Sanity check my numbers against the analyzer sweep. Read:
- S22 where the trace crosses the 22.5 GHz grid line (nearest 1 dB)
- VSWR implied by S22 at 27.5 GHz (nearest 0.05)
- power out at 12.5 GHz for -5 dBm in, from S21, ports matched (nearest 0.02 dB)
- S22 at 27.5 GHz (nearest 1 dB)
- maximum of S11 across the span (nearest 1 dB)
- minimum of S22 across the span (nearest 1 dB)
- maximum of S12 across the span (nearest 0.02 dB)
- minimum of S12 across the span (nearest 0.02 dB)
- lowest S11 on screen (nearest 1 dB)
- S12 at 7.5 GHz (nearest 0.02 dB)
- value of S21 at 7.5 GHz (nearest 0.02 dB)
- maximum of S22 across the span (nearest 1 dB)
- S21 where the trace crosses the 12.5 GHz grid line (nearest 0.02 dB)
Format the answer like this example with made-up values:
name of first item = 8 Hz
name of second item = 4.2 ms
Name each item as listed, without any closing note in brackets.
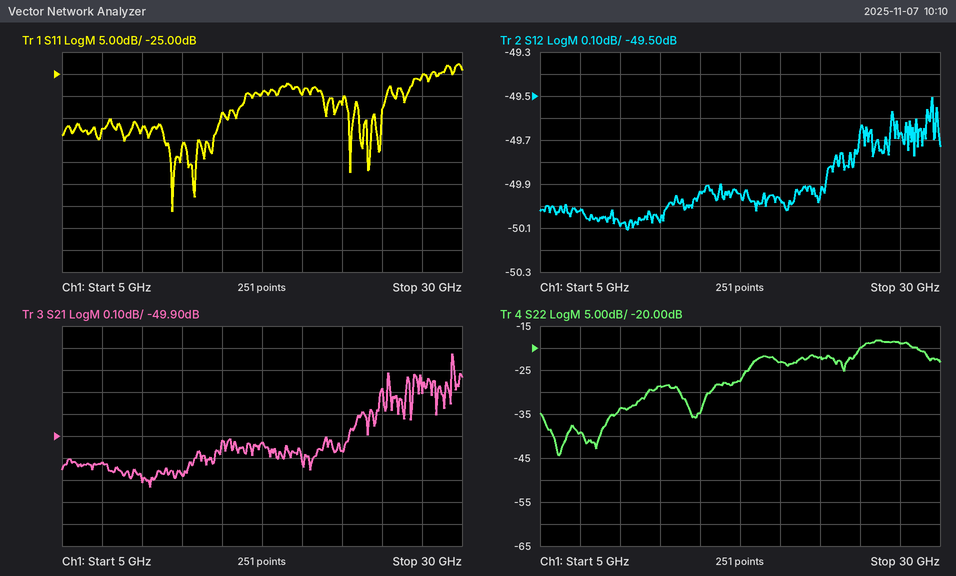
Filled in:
S22 where the trace crosses the 22.5 GHz grid line = -22 dB
VSWR implied by S22 at 27.5 GHz = 1.25
power out at 12.5 GHz for -5 dBm in, from S21, ports matched = -55.08 dBm
S22 at 27.5 GHz = -19 dB
maximum of S11 across the span = -23 dB
minimum of S22 across the span = -44 dB
maximum of S12 across the span = -49.50 dB
minimum of S12 across the span = -50.10 dB
lowest S11 on screen = -56 dB
S12 at 7.5 GHz = -50.02 dB
value of S21 at 7.5 GHz = -50.02 dB
maximum of S22 across the span = -18 dB
S21 where the trace crosses the 12.5 GHz grid line = -50.08 dB
